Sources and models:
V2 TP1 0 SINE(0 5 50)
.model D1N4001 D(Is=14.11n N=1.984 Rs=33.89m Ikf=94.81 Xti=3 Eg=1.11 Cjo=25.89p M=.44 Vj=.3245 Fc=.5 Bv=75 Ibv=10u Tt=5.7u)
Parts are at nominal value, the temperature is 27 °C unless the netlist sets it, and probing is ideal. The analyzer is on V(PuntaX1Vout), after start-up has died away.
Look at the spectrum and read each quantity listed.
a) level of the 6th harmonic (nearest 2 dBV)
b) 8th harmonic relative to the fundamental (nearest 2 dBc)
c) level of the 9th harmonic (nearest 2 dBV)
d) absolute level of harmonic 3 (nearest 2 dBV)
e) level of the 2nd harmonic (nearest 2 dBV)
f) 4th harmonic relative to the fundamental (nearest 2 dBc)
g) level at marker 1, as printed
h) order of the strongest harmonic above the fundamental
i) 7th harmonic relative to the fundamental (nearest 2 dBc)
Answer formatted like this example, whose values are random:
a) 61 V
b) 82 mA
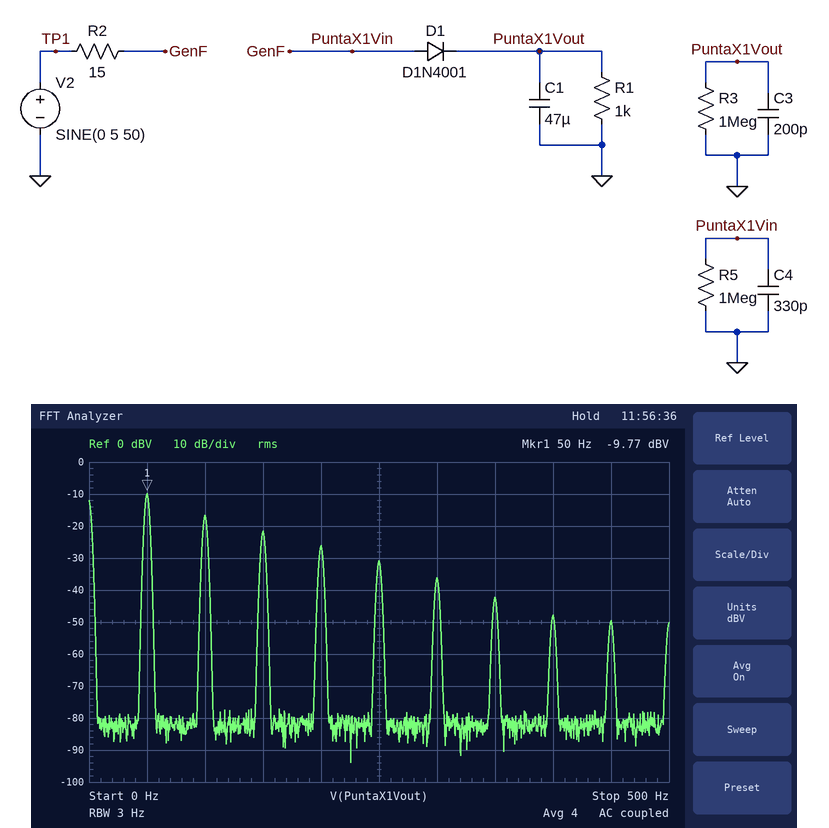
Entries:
a) -36 dBV
b) -38 dBc
c) -50 dBV
d) -22 dBV
e) -16 dBV
f) -16 dBc
g) -9.77 dBV
h) 2
i) -32 dBc
